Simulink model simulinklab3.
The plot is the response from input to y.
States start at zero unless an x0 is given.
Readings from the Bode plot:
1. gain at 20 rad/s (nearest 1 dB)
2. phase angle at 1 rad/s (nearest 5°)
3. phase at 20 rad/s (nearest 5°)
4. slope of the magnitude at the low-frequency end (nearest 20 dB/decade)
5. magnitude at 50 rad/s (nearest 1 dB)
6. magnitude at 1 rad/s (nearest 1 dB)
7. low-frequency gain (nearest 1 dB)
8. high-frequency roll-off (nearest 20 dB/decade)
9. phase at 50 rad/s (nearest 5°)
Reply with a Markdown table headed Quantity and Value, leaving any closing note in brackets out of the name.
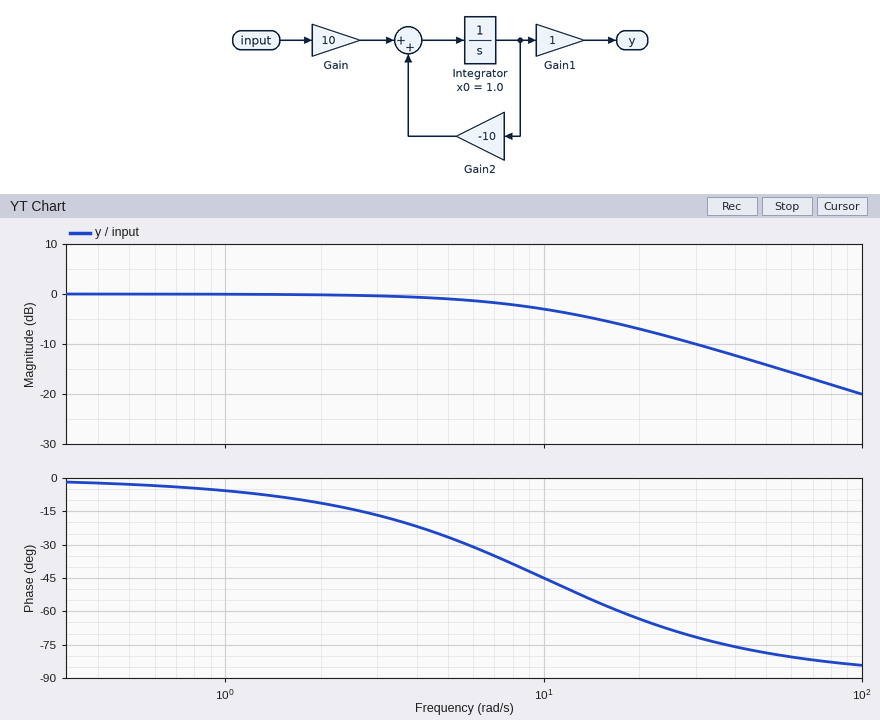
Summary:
| Quantity | Value |
|---|---|
| gain at 20 rad/s | -7 dB |
| phase angle at 1 rad/s | -5° |
| phase at 20 rad/s | -65° |
| slope of the magnitude at the low-frequency end | 0 dB/decade |
| magnitude at 50 rad/s | -14 dB |
| magnitude at 1 rad/s | 0 dB |
| low-frequency gain | 0 dB |
| high-frequency roll-off | -20 dB/decade |
| phase at 50 rad/s | -80° |
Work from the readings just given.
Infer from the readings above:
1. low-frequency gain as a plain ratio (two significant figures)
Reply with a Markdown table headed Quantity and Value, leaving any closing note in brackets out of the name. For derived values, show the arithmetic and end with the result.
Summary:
| Quantity | Value |
|---|---|
| low-frequency gain as a plain ratio | 10^(0 / 20) = 1.0 |
